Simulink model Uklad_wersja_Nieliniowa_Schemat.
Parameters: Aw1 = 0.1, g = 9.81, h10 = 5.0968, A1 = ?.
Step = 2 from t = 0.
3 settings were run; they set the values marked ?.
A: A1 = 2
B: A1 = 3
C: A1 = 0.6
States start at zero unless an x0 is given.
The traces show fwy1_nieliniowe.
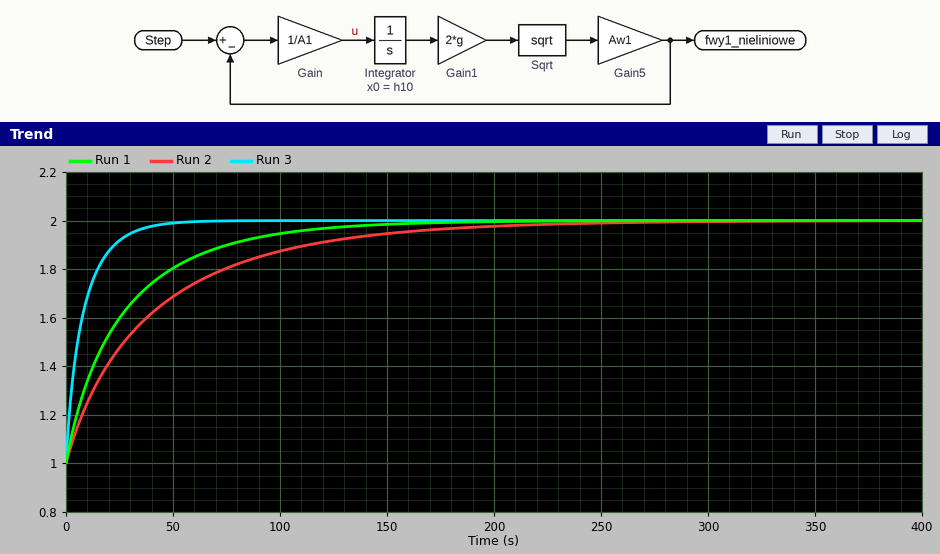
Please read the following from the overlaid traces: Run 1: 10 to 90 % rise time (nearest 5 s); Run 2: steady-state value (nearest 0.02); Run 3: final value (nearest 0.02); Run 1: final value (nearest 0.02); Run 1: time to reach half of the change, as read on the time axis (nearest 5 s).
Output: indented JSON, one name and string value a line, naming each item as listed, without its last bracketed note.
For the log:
{
  "Run 1: 10 to 90 % rise time": "75 s",
  "Run 2: steady-state value": "2.00",
  "Run 3: final value": "2.00",
  "Run 1: final value": "2.00",
  "Run 1: time to reach half of the change, as read on the time axis": "20 s"
}
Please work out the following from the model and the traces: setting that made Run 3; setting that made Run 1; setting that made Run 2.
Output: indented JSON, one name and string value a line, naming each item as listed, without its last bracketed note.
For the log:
{
  "setting that made Run 3": "C",
  "setting that made Run 1": "A",
  "setting that made Run 2": "B"
}
